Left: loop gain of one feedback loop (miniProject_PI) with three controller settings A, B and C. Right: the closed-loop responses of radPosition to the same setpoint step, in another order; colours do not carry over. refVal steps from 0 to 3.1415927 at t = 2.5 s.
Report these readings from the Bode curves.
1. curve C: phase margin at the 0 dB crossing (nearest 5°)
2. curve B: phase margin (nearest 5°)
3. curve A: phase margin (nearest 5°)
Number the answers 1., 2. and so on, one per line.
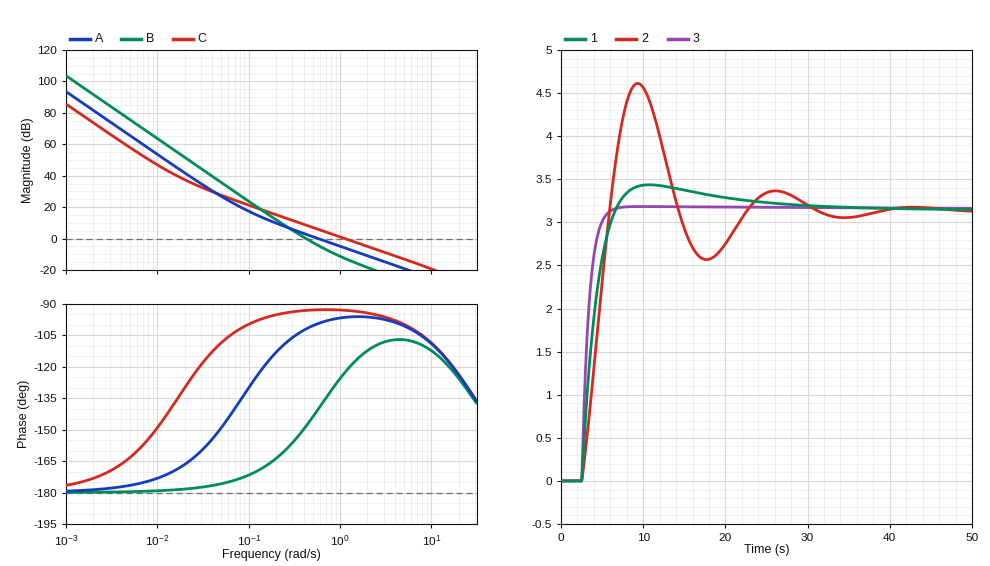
1. 85°
2. 30°
3. 80°
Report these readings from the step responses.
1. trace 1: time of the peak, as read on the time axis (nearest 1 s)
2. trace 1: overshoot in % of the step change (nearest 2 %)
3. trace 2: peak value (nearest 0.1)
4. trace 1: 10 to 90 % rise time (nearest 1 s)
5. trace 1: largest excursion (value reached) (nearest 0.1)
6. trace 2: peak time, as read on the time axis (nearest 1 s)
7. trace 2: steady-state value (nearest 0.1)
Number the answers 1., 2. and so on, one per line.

1. 11 s
2. 10 %
3. 4.6
4. 3 s
5. 3.4
6. 9 s
7. 3.1
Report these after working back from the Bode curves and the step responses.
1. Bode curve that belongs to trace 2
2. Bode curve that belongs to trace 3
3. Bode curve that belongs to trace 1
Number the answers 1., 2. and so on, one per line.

1. B
2. C
3. A
